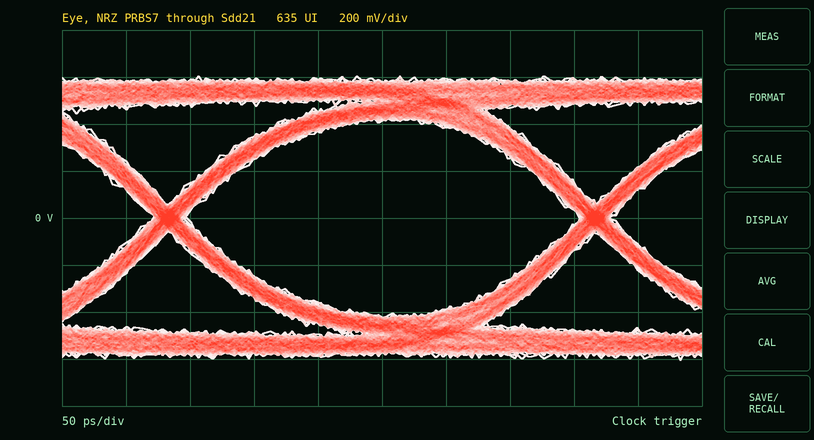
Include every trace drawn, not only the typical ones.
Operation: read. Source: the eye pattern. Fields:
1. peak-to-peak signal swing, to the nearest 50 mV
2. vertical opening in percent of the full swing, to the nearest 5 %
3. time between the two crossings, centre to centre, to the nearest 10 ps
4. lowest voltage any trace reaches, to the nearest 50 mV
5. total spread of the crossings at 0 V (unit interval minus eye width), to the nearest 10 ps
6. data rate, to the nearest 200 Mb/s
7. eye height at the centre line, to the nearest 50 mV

1.20 V
70 %
330 ps
-600 mV
30 ps
3.0 Gb/s
850 mV
